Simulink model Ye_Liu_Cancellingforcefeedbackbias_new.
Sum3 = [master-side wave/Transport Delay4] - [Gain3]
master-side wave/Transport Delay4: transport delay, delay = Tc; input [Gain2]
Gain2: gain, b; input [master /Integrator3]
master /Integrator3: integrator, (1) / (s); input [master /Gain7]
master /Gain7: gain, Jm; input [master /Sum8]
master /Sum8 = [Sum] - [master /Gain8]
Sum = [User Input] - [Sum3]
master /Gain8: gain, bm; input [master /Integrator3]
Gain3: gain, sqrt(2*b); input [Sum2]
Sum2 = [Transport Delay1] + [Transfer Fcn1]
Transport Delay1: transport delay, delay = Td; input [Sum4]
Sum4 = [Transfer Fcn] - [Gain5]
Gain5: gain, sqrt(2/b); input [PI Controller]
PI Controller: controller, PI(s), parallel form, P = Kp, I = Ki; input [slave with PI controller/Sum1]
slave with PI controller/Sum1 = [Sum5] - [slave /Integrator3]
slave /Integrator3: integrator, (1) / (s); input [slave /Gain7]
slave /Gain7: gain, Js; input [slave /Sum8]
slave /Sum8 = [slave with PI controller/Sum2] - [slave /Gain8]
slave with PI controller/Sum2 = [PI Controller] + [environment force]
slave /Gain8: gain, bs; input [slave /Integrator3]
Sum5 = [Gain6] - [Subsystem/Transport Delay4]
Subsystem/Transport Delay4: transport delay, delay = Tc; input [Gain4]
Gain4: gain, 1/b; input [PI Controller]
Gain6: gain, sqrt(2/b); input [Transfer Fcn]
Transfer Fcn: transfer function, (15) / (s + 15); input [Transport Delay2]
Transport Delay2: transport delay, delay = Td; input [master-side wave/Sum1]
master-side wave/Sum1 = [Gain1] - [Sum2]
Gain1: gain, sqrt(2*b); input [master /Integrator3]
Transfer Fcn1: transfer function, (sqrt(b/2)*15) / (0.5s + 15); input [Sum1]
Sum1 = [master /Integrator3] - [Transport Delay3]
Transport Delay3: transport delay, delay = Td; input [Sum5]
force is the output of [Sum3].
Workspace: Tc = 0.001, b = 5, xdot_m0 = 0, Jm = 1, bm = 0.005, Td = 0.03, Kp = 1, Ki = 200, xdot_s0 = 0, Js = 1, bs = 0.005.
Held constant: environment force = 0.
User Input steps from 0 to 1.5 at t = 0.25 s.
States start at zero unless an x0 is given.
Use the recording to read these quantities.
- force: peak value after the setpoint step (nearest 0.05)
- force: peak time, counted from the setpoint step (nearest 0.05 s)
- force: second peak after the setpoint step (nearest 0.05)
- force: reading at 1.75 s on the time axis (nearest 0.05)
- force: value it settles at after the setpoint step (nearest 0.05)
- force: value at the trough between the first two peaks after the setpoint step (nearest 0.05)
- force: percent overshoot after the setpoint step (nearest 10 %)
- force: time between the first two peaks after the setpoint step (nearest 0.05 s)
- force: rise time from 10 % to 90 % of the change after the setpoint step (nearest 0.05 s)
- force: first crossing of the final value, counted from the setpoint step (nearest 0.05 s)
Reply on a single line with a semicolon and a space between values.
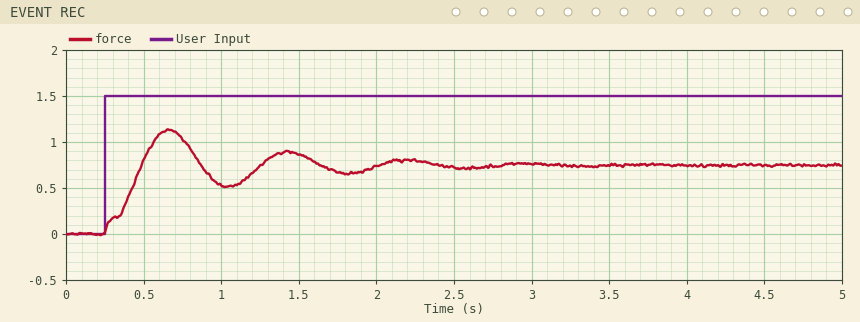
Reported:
1.15; 0.40 s; 0.90; 0.65; 0.75; 0.50; 50 %; 0.75 s; 0.20 s; 0.25 s
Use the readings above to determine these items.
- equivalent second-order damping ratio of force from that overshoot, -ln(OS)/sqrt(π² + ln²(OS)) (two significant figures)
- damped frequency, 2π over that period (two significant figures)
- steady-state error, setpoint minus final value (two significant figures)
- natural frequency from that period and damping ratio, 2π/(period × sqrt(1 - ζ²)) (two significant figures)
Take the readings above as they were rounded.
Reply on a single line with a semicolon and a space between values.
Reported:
0.22; 8.4 rad/s; 0.75; 8.6 rad/s
